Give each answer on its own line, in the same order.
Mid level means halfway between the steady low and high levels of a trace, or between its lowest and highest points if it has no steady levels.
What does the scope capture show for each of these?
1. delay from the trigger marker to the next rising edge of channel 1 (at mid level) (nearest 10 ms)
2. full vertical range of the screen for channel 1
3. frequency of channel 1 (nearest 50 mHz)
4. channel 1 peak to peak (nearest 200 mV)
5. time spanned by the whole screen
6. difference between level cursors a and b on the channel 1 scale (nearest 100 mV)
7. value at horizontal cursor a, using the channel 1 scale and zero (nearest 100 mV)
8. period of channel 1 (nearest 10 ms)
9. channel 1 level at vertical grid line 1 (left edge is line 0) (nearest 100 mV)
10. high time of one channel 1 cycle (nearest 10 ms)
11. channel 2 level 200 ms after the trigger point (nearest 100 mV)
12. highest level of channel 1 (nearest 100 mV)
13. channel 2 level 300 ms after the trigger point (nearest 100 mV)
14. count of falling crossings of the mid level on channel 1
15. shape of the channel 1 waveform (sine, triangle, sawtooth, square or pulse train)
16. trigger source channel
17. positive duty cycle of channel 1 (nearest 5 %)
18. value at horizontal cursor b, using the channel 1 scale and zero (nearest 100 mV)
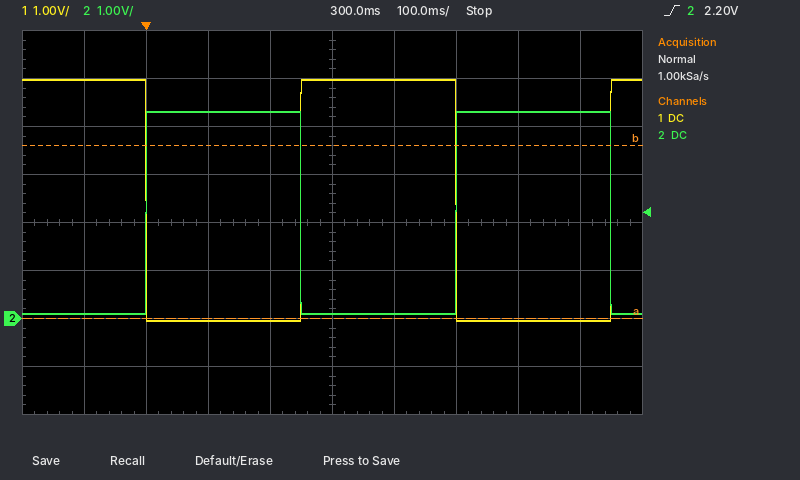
250 ms
8 V
2.00 Hz
5.0 V
1 s
3.6 V
0.0 V
500 ms
5.0 V
250 ms
4.3 V
5.0 V
100 mV
2
square
channel 2
50 %
3.6 V
